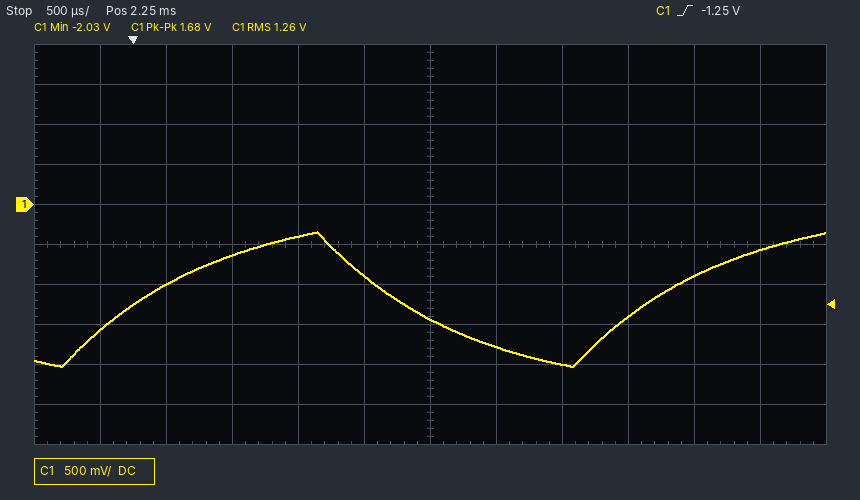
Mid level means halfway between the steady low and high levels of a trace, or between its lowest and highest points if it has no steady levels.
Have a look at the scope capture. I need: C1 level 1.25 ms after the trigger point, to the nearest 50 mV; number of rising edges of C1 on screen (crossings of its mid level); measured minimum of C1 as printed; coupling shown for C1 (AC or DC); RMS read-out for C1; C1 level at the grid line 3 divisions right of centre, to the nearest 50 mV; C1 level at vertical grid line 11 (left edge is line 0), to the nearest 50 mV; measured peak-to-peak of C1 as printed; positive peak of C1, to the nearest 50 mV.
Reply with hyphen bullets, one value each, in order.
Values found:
- -400 mV
- 2
- -2.03 V
- DC
- 1.26 V
- -1.40 V
- -550 mV
- 1.68 V
- -350 mV
